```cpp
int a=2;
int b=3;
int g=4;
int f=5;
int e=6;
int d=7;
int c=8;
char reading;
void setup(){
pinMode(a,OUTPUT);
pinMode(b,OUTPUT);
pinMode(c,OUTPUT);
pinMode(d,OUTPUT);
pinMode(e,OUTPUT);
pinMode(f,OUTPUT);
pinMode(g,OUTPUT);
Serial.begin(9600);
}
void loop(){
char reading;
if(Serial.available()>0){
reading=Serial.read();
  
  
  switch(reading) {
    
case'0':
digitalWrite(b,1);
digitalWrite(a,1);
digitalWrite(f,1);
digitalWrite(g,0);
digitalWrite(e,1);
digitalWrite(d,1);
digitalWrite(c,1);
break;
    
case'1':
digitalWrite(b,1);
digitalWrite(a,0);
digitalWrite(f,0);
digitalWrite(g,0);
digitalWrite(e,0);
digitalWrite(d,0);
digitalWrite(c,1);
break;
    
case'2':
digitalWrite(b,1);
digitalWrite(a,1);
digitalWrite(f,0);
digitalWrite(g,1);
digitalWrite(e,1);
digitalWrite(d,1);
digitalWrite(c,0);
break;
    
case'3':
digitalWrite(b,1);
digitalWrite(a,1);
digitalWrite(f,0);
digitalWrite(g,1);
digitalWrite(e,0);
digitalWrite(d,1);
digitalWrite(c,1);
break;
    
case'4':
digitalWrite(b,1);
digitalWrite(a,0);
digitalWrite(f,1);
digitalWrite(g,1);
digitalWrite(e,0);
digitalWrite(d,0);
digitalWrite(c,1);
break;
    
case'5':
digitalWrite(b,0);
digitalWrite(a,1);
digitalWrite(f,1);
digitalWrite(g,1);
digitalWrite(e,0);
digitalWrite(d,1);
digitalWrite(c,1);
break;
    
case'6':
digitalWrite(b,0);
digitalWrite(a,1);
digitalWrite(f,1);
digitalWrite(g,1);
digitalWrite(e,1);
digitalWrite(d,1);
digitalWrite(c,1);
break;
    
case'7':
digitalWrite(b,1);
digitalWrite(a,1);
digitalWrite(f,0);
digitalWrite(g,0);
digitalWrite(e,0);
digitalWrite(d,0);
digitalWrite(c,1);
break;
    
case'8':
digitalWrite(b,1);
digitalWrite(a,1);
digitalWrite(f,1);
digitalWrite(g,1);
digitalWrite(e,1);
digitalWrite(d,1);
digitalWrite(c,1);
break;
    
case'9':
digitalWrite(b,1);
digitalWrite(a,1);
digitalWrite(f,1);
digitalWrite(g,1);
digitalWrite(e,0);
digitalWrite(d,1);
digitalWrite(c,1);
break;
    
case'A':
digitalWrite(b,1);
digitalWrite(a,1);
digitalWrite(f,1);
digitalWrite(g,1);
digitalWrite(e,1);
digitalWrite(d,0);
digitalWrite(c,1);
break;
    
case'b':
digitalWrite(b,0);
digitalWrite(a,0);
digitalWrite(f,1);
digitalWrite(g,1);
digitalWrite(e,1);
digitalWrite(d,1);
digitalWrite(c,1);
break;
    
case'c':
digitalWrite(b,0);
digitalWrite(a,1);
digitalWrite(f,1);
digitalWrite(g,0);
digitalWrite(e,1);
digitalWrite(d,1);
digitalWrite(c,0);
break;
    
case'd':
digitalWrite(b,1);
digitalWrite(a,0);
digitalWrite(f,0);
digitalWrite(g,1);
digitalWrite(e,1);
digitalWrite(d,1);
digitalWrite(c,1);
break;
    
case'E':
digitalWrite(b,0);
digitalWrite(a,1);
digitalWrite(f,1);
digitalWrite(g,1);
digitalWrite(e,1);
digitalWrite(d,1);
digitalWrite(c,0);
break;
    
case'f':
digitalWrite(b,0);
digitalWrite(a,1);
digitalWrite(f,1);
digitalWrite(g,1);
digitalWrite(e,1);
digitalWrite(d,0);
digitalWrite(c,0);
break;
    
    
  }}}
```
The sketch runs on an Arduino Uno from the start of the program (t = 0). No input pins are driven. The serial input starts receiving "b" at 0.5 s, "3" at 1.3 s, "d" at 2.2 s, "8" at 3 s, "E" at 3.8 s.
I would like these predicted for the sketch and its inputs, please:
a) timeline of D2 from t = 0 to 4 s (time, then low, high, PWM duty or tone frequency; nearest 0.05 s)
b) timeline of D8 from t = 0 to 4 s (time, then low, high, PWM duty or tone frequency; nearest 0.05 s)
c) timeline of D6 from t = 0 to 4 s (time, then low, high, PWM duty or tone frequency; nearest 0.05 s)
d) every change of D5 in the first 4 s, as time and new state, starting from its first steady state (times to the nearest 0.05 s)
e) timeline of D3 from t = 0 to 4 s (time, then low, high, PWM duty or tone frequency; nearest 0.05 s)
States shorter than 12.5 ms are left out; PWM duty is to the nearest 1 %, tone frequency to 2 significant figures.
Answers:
0 s low; 1.3 s high; 2.2 s low; 3 s high
0 s low; 0.5 s high; 3.8 s low
0 s low; 0.5 s high; 1.3 s low; 2.2 s high
0 s low; 0.5 s high; 1.3 s low; 3 s high
0 s low; 1.3 s high; 3.8 s low
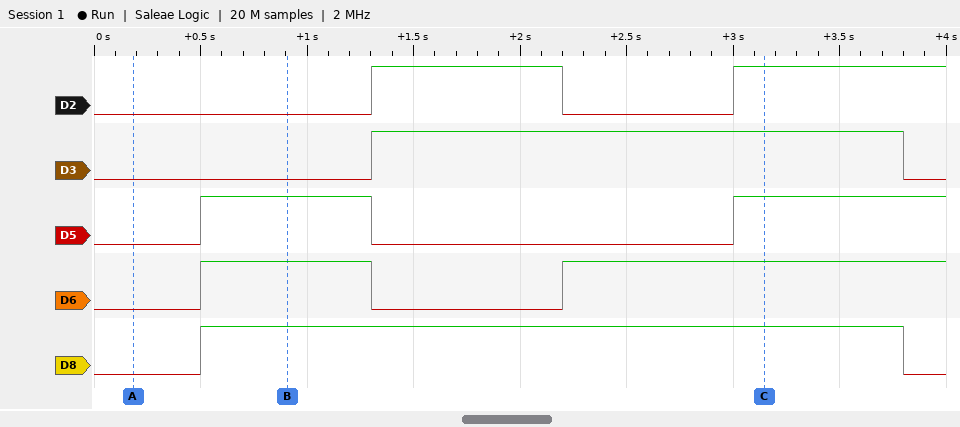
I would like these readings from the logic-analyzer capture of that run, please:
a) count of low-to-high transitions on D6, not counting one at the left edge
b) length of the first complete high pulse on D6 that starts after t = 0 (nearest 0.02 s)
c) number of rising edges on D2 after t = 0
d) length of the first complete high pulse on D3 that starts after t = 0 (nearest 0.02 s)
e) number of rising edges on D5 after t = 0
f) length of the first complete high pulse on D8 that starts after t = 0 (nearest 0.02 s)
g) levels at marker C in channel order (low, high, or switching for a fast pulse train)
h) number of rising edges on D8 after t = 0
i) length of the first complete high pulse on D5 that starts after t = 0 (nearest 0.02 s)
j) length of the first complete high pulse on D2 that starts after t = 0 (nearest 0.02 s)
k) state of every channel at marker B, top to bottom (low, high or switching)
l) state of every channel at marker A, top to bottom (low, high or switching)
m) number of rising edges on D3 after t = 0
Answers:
2
0.80 s
2
2.50 s
2
3.30 s
D2 high, D3 high, D5 high, D6 high, D8 high
1
0.80 s
0.90 s
D2 low, D3 low, D5 high, D6 high, D8 high
D2 low, D3 low, D5 low, D6 low, D8 low
1
